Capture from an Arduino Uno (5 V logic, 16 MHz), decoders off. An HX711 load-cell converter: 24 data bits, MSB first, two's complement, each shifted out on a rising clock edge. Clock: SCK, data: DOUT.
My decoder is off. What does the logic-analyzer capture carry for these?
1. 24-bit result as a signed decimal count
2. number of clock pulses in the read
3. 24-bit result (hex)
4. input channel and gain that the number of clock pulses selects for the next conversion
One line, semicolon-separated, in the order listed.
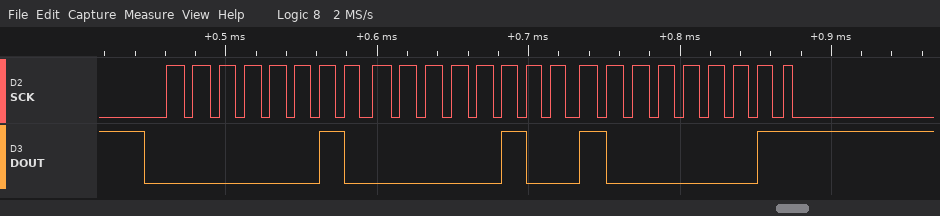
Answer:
132225; 25; 0x020481; channel A, gain 128
